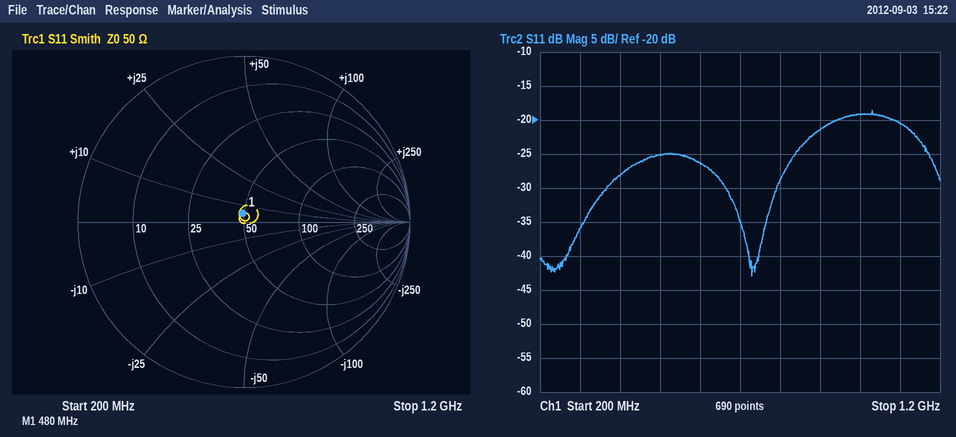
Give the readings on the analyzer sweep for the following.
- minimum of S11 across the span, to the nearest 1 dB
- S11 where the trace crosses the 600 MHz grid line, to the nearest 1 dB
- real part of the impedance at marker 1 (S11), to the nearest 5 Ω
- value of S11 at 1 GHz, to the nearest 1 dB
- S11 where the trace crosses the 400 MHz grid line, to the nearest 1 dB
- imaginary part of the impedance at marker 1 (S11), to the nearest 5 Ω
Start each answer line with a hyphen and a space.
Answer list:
- -43 dB
- -26 dB
- 50 Ω
- -19 dB
- -28 dB
- +5 Ω
